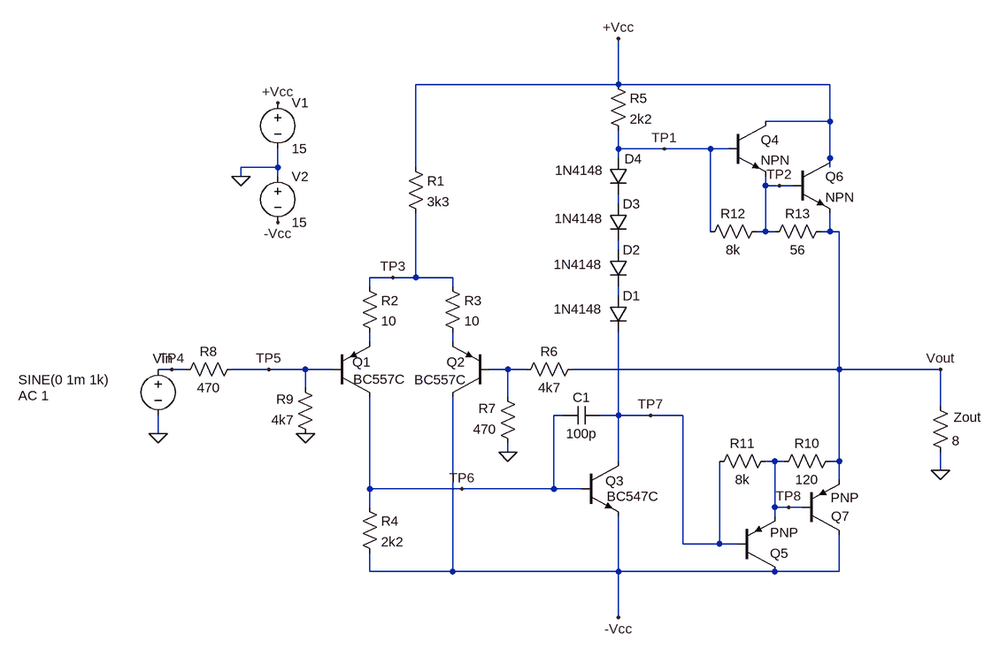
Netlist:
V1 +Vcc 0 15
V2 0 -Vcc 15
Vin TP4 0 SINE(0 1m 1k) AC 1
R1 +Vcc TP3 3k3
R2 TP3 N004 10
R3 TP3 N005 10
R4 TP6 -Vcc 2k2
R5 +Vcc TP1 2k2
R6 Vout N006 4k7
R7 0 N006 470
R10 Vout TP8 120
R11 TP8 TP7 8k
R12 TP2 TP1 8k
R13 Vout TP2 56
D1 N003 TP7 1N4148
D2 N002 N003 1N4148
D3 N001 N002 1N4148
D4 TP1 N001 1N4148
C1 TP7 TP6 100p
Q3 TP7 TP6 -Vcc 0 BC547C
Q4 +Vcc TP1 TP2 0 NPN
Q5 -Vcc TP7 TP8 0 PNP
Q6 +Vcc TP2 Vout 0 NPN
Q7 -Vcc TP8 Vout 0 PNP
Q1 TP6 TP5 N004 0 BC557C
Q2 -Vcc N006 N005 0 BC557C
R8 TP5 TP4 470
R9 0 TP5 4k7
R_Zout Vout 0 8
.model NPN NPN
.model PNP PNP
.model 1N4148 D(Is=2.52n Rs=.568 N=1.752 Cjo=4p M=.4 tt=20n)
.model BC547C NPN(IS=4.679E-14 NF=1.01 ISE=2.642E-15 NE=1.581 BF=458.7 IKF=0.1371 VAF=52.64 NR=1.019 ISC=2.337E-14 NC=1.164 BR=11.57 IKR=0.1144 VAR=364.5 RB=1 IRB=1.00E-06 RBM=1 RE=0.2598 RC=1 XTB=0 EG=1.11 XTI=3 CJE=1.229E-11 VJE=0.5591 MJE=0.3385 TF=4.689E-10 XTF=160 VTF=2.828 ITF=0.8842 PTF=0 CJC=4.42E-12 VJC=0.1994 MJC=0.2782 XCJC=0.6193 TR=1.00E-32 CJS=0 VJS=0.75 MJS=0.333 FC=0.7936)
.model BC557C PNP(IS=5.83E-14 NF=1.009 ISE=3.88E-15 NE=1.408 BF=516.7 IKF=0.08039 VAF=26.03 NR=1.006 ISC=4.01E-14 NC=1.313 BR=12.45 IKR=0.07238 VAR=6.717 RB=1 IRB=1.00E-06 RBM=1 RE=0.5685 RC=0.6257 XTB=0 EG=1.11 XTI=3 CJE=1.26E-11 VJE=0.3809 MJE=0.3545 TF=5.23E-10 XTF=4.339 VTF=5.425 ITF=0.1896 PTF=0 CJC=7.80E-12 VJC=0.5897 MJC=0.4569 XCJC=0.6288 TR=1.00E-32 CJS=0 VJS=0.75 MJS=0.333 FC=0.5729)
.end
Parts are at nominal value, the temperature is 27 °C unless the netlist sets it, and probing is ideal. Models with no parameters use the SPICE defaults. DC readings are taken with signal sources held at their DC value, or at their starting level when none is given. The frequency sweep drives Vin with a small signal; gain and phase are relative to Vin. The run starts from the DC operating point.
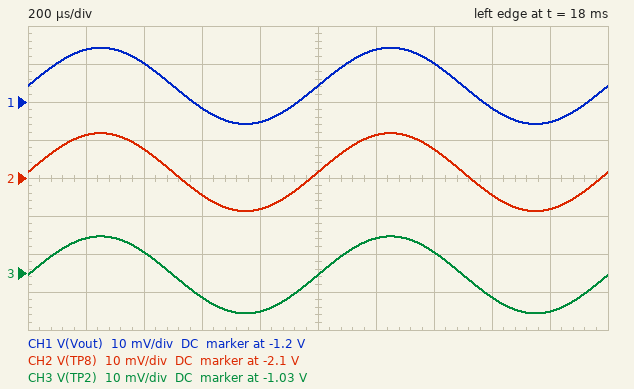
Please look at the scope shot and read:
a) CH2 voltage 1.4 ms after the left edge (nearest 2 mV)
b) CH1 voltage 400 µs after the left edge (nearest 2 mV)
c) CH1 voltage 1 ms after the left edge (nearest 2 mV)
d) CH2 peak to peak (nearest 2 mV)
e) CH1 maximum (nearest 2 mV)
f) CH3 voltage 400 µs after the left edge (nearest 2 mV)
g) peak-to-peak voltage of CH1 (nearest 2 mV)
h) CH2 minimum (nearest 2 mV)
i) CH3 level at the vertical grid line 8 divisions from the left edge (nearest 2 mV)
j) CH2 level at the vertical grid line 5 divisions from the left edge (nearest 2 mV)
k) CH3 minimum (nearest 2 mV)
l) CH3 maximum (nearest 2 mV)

-2.092 V
-1.190 V
-1.196 V
20 mV
-1.186 V
-1.024 V
20 mV
-2.108 V
-1.036 V
-2.098 V
-1.040 V
-1.020 V
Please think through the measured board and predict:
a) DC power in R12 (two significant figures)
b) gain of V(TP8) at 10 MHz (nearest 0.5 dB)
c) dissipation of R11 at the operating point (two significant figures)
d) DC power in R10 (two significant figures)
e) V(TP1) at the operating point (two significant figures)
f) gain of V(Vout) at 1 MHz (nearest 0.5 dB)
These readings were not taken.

80 µW
-0.5 dB
86 µW
6.8 mW
-230 mV
18.5 dB
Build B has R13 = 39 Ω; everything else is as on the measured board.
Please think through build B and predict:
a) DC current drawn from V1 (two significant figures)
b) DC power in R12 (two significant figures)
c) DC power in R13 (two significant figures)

15 mA
82 µW
630 µW
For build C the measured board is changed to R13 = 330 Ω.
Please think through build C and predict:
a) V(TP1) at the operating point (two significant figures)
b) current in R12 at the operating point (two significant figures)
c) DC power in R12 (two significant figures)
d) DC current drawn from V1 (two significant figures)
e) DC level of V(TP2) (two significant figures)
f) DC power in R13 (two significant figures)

-230 mV
95 µA
72 µW
12 mA
-990 mV
130 µW
